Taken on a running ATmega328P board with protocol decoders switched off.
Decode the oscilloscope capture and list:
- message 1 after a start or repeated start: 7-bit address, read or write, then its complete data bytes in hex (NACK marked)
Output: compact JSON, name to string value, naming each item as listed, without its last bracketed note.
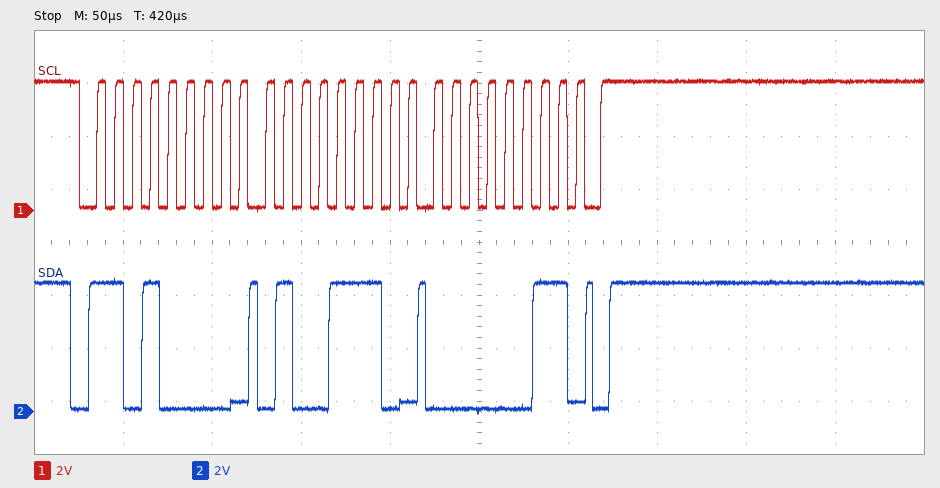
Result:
{"message 1 after a start or repeated start: 7-bit address, read or write, then its complete data bytes in hex": "0x68 write: 4E 03"}
